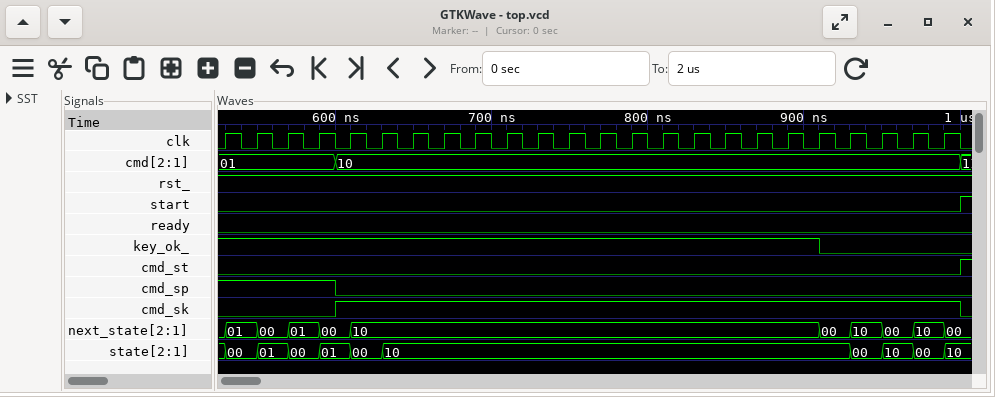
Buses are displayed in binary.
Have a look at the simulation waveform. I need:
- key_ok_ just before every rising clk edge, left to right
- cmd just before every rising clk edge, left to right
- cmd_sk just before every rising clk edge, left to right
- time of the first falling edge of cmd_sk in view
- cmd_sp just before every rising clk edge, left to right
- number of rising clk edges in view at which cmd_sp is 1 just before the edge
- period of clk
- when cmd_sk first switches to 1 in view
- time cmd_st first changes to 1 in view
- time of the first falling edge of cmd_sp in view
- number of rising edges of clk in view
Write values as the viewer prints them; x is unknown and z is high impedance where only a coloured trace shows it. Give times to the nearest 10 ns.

1 1 1 1 1 1 1 1 1 1 1 1 1 1 1 1 1 1 1 1 0 0 0 0
01, 01, 01, 01, 10, 10, 10, 10, 10, 10, 10, 10, 10, 10, 10, 10, 10, 10, 10, 10, 10, 10, 10, 10
0 0 0 0 1 1 1 1 1 1 1 1 1 1 1 1 1 1 1 1 1 1 1 1
1000 ns
1 1 1 1 0 0 0 0 0 0 0 0 0 0 0 0 0 0 0 0 0 0 0 0
4
20 ns
600 ns
1000 ns
600 ns
24
